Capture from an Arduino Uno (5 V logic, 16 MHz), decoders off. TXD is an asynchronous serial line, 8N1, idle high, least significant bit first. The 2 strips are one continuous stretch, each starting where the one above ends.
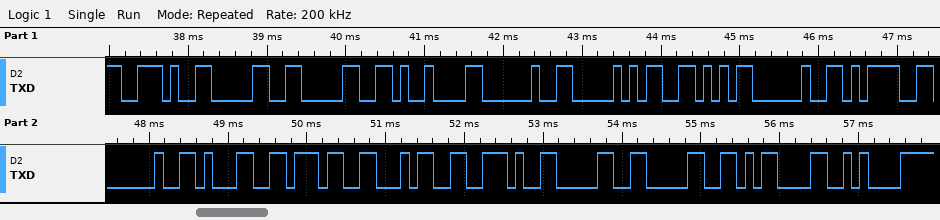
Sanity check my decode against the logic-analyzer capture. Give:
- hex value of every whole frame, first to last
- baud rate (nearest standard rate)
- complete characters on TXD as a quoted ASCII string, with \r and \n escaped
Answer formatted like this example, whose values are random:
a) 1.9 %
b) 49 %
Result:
a) 0x2E 0x30 0x30 0x09 0x20 0x50 0x56 0x20 0x3D 0x20 0x31 0x37 0x34 0x2E 0x30 0x30 0x0D 0x0A
b) 9600 baud
c) ".00\t PV = 174.00\r\n"
